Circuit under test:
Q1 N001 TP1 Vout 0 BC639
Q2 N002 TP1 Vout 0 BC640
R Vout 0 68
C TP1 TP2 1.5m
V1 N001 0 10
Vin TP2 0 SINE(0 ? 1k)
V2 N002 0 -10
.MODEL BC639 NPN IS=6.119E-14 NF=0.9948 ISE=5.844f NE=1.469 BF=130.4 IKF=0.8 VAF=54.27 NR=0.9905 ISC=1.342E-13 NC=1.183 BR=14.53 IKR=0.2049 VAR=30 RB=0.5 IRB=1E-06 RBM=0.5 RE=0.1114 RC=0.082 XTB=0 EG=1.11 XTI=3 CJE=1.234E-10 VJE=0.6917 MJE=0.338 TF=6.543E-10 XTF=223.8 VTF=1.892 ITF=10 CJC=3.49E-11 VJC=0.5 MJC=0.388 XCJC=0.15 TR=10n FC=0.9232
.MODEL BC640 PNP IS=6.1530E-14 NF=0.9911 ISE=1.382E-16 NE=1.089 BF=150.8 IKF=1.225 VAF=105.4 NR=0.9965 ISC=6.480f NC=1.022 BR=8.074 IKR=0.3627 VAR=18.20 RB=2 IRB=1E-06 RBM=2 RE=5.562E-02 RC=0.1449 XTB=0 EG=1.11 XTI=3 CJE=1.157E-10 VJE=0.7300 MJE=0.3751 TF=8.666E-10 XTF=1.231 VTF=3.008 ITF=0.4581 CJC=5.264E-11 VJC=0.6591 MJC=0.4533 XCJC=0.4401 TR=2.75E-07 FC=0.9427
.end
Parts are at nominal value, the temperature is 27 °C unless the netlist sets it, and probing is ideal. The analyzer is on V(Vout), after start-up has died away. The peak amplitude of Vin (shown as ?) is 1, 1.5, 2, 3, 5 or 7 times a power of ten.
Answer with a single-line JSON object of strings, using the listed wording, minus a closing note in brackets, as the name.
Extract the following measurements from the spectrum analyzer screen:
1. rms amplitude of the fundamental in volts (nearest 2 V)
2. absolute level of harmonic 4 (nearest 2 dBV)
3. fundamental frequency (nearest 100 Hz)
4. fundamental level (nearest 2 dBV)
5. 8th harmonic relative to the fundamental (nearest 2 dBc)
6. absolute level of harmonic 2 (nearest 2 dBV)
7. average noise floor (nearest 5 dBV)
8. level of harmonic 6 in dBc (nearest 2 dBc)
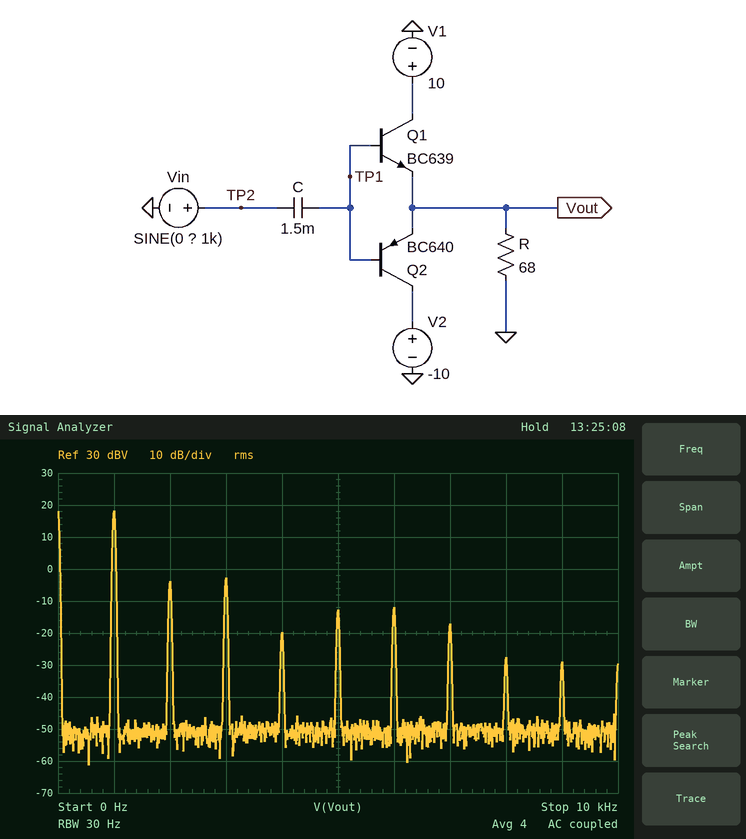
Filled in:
{"rms amplitude of the fundamental in volts": "8 V", "absolute level of harmonic 4": "-20 dBV", "fundamental frequency": "1.0 kHz", "fundamental level": "18 dBV", "8th harmonic relative to the fundamental": "-46 dBc", "absolute level of harmonic 2": "-4 dBV", "average noise floor": "-50 dBV", "level of harmonic 6 in dBc": "-30 dBc"}
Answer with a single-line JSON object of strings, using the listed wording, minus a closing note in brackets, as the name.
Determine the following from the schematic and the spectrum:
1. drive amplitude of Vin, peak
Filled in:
{"drive amplitude of Vin, peak": "15 V"}
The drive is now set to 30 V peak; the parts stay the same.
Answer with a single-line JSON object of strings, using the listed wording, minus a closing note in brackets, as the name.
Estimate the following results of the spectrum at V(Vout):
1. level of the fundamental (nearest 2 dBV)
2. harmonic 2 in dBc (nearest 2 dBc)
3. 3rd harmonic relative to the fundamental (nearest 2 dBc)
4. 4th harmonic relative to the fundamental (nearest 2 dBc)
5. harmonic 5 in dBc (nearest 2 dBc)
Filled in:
{"level of the fundamental": "20 dBV", "harmonic 2 in dBc": "-14 dBc", "3rd harmonic relative to the fundamental": "-16 dBc", "4th harmonic relative to the fundamental": "-18 dBc", "harmonic 5 in dBc": "-32 dBc"}
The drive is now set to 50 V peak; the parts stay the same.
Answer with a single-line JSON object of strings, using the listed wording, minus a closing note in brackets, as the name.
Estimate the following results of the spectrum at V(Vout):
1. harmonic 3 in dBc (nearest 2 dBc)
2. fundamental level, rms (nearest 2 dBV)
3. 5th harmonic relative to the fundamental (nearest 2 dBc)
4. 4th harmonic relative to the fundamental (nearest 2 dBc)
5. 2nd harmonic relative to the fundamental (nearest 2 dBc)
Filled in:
{"harmonic 3 in dBc": "-18 dBc", "fundamental level, rms": "20 dBV", "5th harmonic relative to the fundamental": "-46 dBc", "4th harmonic relative to the fundamental": "-16 dBc", "2nd harmonic relative to the fundamental": "-12 dBc"}
